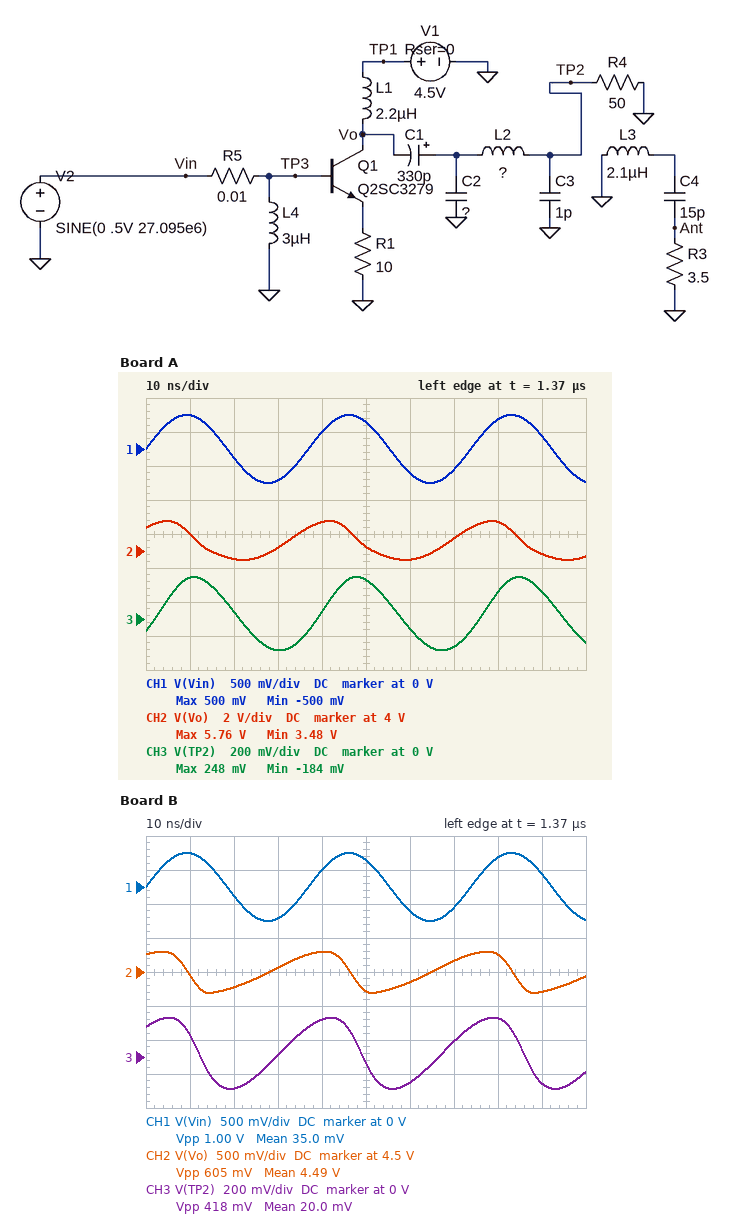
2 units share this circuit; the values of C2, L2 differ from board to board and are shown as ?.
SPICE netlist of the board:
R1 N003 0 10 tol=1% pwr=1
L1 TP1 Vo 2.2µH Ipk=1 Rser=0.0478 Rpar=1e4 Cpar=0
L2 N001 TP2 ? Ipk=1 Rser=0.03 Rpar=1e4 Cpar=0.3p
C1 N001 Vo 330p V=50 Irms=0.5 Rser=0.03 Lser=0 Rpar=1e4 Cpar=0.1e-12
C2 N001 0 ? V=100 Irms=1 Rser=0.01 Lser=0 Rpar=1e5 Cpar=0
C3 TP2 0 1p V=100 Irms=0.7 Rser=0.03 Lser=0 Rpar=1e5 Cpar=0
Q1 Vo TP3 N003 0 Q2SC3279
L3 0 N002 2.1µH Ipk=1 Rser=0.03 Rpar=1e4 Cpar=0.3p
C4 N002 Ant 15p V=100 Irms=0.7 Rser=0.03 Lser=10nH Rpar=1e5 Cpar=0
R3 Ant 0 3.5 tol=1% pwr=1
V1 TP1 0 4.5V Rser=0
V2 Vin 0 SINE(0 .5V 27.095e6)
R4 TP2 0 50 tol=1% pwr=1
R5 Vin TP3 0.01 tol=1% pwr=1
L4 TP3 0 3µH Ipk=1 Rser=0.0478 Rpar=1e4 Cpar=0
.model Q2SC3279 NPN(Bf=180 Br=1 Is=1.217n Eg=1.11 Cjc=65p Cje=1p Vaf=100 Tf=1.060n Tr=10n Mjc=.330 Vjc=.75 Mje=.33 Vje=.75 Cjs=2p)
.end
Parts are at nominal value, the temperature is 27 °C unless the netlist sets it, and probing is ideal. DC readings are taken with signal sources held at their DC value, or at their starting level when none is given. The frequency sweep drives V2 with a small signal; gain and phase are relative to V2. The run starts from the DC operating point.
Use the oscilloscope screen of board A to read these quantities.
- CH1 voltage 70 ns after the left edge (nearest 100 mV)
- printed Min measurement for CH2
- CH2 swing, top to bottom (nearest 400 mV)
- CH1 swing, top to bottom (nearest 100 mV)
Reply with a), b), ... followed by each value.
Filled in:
a) -300 mV
b) 3.48 V
c) 2.4 V
d) 1.0 V
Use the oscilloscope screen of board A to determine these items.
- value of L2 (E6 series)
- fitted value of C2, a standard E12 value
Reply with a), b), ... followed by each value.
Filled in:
a) 1.5 µH
b) 22 pF
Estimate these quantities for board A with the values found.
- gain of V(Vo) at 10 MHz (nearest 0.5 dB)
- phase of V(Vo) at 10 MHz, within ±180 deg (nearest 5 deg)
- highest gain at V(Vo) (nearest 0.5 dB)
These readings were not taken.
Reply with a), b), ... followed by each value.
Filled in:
a) -17.0 dB
b) 145 deg
c) 10.5 dB
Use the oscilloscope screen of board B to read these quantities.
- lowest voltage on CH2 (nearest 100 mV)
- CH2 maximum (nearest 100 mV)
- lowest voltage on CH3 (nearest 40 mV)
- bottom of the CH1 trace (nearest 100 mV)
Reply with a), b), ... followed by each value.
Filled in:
a) 4.2 V
b) 4.8 V
c) -200 mV
d) -500 mV
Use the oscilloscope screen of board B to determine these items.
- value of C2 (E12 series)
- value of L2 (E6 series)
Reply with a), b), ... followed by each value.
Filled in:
a) 82 pF
b) 220 nH
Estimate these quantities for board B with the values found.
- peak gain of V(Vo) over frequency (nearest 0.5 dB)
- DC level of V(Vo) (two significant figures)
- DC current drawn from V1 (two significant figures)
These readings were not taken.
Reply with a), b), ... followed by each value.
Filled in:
a) -7.0 dB
b) 4.5 V
c) 450 µA
